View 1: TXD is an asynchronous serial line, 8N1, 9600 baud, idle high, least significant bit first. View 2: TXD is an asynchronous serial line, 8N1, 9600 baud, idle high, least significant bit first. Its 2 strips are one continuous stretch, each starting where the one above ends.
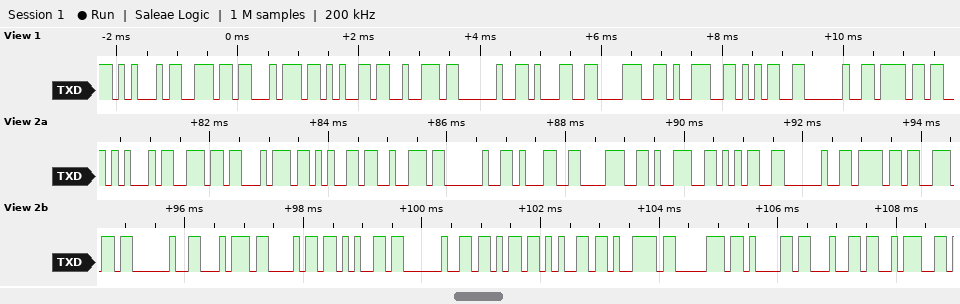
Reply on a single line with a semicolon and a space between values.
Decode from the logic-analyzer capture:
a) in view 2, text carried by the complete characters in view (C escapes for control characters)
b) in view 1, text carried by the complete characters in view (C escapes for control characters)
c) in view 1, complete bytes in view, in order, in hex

"Enter 1895 on the keypad:"; "Enter 1895 o"; 0x45 0x6E 0x74 0x65 0x72 0x20 0x31 0x38 0x39 0x35 0x20 0x6F
